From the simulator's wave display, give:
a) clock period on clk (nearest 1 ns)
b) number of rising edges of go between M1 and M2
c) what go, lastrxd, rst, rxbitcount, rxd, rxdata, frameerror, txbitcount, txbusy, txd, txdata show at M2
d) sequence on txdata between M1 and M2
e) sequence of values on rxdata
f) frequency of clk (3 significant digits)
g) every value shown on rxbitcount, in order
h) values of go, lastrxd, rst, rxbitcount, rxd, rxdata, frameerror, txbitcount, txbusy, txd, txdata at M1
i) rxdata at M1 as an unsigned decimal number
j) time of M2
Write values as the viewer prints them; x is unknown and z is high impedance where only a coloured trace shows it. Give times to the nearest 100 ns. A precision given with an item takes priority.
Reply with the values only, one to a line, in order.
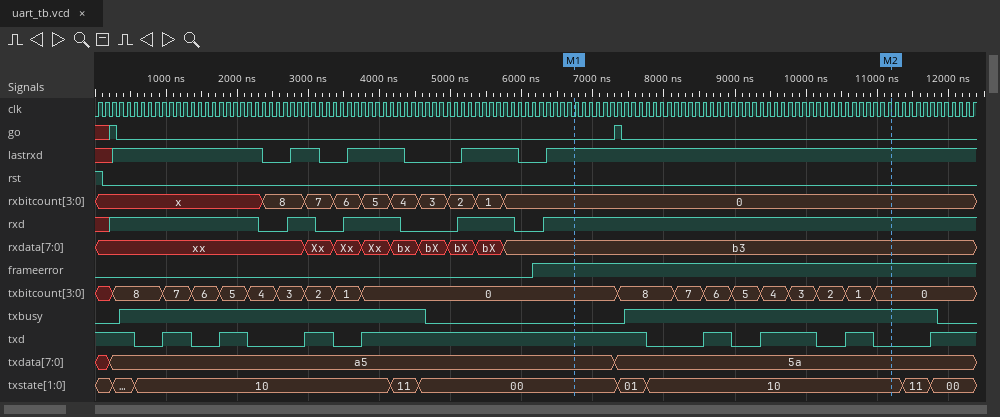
100 ns
1
go=0, lastrxd=1, rst=0, rxbitcount=0, rxd=1, rxdata=b3, frameerror=1, txbitcount=0, txbusy=1, txd=0, txdata=5a
a5, 5a
xx, Xx, Xx, Xx, bx, bX, bX, bX, b3
10.0 MHz
x, 8, 7, 6, 5, 4, 3, 2, 1, 0
go=0, lastrxd=1, rst=0, rxbitcount=0, rxd=1, rxdata=b3, frameerror=1, txbitcount=0, txbusy=0, txd=1, txdata=a5
179
11200 ns
